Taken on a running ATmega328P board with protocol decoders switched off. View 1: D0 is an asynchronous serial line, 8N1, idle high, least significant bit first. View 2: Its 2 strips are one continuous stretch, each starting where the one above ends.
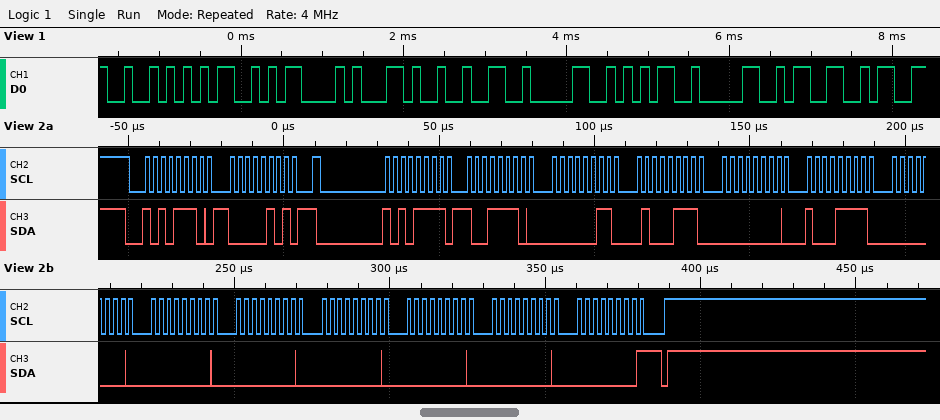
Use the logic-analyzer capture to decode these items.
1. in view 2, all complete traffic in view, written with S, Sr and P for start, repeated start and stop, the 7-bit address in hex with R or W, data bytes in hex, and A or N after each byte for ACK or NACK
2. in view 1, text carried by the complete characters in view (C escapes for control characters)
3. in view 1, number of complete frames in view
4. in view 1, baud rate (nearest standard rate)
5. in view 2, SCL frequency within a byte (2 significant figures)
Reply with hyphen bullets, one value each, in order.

- S 57W A 05 A Sr 57R A 9E A 03 A 47 A 00 A 8F A 00 A 00 A 00 A 00 A 00 A 00 A 00 N P
- "RMC,20503"
- 9
- 9600 baud
- 400 kHz
